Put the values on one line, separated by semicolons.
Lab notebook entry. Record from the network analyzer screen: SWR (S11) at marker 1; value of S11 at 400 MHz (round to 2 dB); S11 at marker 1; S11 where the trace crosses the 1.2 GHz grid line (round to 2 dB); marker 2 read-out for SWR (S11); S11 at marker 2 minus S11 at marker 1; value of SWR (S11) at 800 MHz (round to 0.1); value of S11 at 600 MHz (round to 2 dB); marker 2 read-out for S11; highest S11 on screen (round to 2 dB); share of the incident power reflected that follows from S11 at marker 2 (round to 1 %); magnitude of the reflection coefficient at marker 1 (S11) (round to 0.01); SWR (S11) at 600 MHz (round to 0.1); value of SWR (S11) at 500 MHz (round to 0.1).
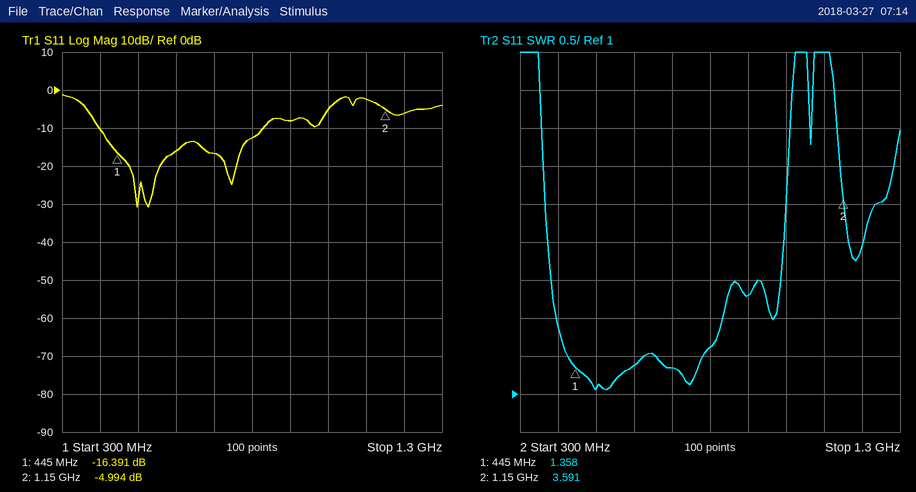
1.358; -10 dB; -16.391 dB; -6 dB; 3.591; 11.397 dB; 1.6; -16 dB; -4.994 dB; -2 dB; 32 %; 0.15; 1.4; 1.1
